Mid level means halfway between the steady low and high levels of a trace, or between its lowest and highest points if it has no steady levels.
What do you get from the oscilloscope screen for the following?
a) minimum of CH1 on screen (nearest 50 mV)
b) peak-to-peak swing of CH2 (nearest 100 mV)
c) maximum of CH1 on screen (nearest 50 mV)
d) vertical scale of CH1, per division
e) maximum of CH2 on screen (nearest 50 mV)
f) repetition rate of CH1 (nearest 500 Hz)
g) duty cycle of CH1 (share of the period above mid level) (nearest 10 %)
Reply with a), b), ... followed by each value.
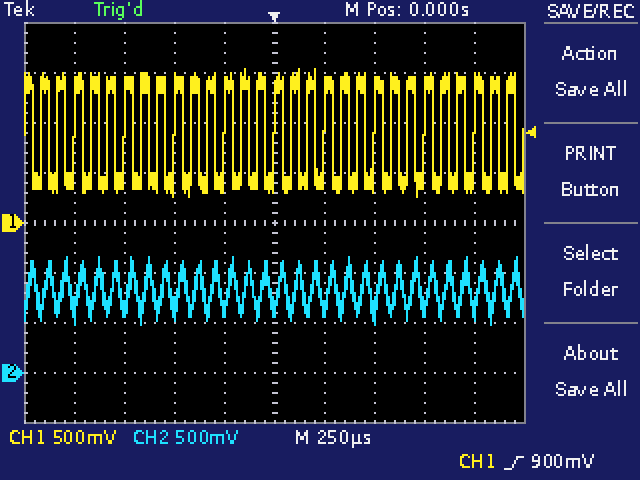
a) 250 mV
b) 700 mV
c) 1.55 V
d) 500 mV
e) 1.15 V
f) 12.0 kHz
g) 50 %
